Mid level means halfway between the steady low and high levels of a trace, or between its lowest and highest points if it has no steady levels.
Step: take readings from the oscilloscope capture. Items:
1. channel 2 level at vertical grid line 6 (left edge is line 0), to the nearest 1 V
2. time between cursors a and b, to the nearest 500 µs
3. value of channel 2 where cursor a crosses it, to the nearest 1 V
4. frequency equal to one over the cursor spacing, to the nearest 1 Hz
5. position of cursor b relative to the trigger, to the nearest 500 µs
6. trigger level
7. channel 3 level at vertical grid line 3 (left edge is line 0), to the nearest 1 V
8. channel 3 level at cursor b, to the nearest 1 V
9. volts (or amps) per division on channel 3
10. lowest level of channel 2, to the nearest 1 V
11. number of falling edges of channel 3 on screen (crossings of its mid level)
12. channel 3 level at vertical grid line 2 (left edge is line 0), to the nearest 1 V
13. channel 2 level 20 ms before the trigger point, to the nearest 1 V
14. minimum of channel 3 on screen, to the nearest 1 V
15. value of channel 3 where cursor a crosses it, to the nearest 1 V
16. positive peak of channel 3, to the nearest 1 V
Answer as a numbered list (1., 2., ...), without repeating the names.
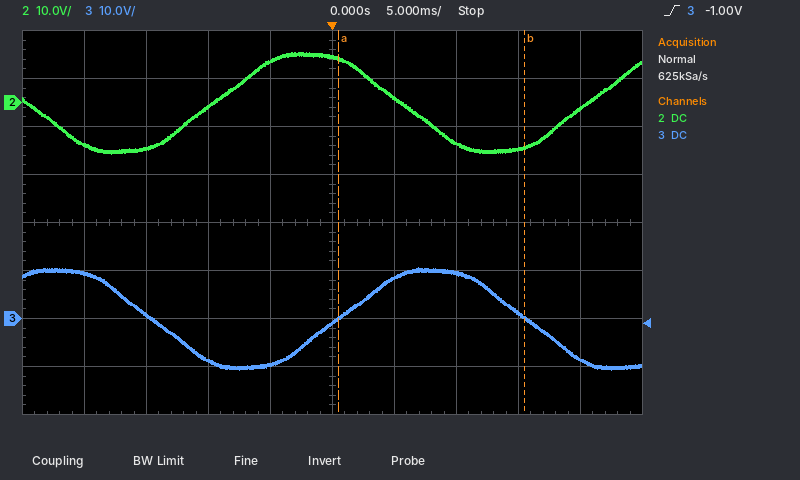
1. 1 V
2. 15.0 ms
3. 9 V
4. 67 Hz
5. +15.5 ms
6. -1.00 V
7. -9 V
8. 0 V
9. 10 V
10. -11 V
11. 2
12. 1 V
13. -9 V
14. -11 V
15. 0 V
16. 11 V
